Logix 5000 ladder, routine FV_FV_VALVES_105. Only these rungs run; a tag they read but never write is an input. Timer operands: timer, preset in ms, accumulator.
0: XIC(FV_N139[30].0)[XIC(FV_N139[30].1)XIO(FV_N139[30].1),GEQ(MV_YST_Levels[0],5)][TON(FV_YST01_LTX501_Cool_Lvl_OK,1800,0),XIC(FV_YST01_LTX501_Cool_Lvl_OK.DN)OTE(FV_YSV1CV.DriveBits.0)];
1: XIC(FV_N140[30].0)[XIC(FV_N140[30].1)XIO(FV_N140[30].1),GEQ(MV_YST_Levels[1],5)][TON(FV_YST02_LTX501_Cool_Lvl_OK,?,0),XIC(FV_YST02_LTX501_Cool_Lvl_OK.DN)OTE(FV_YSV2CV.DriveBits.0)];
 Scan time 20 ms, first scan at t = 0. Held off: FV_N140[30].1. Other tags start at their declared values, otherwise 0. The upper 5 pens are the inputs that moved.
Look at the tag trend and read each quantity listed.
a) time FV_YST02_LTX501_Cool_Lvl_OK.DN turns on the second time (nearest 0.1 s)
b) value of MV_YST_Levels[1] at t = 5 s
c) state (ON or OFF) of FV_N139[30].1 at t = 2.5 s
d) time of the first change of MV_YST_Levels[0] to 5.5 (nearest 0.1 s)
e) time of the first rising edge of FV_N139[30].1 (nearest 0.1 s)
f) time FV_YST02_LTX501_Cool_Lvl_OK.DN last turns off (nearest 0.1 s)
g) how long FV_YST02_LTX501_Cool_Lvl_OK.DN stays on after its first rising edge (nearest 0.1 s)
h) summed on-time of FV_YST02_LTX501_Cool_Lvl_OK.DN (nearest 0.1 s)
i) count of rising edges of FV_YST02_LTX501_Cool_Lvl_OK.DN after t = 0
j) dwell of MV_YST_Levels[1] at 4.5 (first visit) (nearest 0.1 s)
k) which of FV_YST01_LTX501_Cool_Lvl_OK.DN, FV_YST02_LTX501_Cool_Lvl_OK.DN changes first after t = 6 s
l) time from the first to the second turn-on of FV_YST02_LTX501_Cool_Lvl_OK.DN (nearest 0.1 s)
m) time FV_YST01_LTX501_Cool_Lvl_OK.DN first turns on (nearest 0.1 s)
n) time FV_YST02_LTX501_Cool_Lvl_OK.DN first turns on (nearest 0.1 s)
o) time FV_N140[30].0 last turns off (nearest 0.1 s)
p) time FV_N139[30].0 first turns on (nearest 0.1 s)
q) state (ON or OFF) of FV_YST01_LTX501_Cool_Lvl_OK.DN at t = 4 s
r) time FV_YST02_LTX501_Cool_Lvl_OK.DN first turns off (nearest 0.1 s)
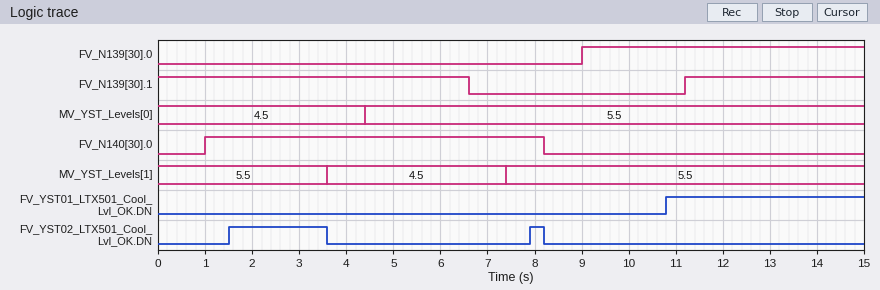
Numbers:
7.9 s
4.5
ON
4.4 s
11.2 s
8.2 s
2.1 s
2.4 s
2
3.8 s
FV_YST02_LTX501_Cool_Lvl_OK.DN
6.4 s
10.8 s
1.5 s
8.2 s
9.0 s
OFF
3.6 s
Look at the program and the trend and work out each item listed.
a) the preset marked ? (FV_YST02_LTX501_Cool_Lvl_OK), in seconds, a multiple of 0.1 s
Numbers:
0.5 s
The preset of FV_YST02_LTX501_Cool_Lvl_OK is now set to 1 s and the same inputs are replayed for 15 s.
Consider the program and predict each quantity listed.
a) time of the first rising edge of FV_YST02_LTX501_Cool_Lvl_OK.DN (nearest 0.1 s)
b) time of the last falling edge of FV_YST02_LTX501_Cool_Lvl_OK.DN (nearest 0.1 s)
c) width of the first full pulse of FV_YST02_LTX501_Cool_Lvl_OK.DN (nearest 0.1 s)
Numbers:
2.0 s
3.6 s
1.6 s
